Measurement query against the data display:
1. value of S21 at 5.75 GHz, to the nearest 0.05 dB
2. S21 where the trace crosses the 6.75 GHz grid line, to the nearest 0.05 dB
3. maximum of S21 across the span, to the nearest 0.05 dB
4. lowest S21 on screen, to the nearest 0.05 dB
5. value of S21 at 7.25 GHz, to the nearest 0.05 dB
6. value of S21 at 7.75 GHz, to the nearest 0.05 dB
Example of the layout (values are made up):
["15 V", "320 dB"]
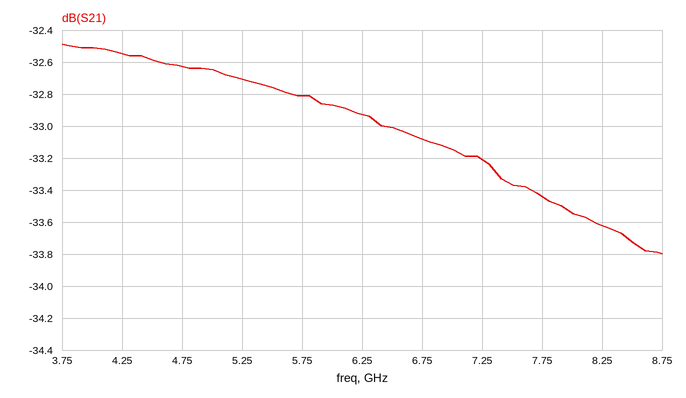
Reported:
["-32.80 dB", "-33.10 dB", "-32.50 dB", "-33.80 dB", "-33.20 dB", "-33.45 dB"]
